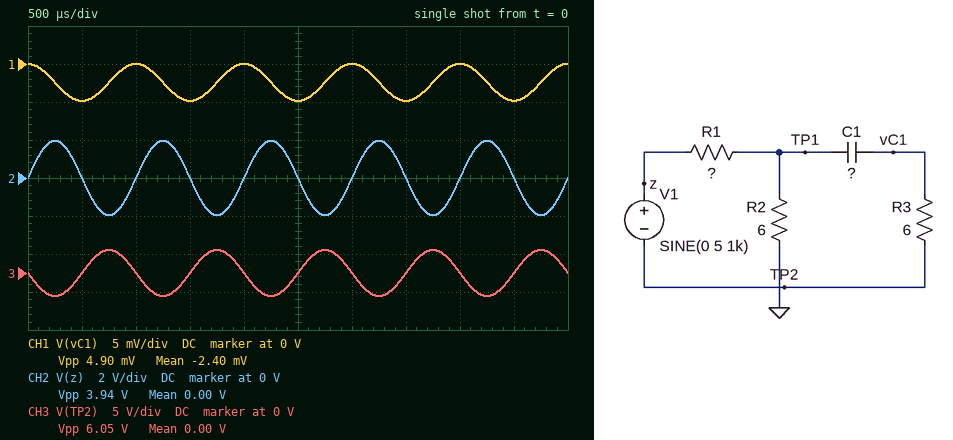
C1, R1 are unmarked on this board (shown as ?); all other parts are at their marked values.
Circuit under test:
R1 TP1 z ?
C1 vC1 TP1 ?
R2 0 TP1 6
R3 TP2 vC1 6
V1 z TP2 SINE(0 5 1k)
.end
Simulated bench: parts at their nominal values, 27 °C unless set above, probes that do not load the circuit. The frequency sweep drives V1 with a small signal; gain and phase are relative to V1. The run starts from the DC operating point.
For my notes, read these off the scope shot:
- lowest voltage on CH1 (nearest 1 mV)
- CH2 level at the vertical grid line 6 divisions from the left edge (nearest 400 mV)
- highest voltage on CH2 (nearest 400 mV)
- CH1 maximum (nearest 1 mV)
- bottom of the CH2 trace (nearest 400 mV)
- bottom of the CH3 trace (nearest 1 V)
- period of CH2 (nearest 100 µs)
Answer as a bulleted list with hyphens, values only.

- -5 mV
- 0 V
- 2.0 V
- 0 V
- -2.0 V
- -3 V
- 1.0 ms
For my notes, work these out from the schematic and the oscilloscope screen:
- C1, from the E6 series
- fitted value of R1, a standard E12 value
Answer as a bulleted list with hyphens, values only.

- 33 mF
- 3.9 Ω
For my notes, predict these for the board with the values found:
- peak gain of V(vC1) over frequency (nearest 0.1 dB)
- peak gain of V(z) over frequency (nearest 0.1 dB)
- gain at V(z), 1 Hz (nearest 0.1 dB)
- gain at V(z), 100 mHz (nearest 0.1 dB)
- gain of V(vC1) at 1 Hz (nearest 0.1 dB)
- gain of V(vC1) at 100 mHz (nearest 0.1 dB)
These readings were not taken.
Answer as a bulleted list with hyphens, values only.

- 0 dB
- -8.1 dB
- -9.0 dB
- -22.0 dB
- -7.2 dB
- -0.2 dB
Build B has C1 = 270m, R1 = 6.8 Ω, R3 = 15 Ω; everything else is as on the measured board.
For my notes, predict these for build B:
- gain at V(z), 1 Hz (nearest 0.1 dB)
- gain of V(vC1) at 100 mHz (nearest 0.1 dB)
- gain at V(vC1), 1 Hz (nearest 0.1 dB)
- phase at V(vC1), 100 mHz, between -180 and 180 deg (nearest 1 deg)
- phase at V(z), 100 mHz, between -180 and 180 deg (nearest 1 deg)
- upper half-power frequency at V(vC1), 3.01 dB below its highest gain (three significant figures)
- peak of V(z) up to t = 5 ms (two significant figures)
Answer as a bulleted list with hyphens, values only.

- -10.1 dB
- -11.7 dB
- -31.4 dB
- 105 deg
- 15 deg
- 27.0 mHz
- 1.6 V
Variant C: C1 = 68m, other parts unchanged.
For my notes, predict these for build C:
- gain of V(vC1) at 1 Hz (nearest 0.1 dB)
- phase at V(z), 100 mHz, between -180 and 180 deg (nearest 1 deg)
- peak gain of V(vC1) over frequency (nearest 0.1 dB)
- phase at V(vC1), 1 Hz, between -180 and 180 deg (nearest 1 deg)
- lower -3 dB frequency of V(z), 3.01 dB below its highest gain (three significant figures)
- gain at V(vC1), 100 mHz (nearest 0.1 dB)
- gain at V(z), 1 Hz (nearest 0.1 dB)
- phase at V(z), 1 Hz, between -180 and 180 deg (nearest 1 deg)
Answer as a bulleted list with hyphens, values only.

- -12.8 dB
- 67 deg
- 0 dB
- 103 deg
- 236 mHz
- -0.7 dB
- -8.3 dB
- 13 deg
